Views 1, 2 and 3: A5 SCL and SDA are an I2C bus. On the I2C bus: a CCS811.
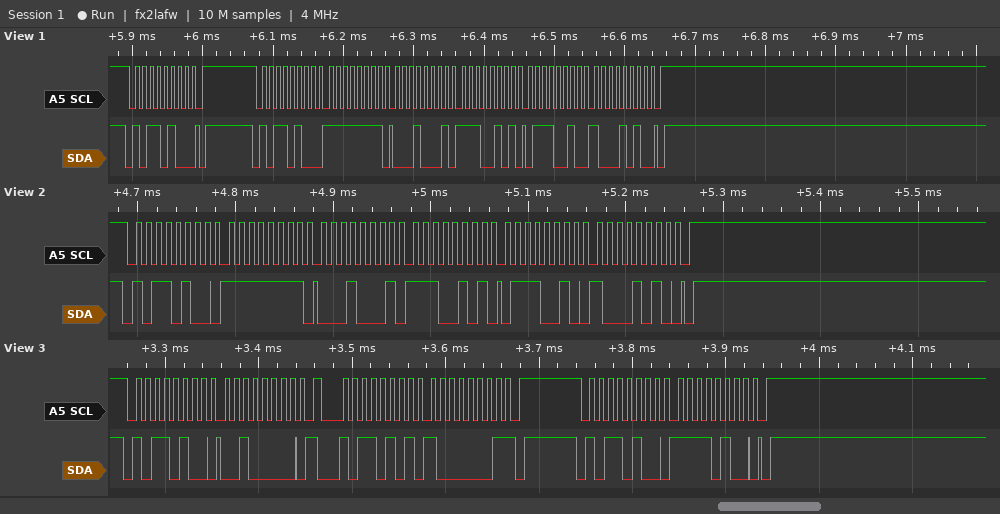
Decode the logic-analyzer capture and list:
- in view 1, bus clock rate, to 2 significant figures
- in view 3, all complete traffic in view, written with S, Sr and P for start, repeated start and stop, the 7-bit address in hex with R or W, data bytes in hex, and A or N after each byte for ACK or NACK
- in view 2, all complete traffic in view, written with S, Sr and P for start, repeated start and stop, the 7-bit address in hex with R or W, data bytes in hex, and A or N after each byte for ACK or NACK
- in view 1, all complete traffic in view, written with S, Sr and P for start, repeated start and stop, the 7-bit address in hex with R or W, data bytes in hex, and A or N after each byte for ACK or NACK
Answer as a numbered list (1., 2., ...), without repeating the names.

1. 100 kHz
2. S 5AW A 20 A Sr 5AR A 81 N P S 5AW A F4 A P
3. S 5AW A FF A 11 A E5 A 72 A 8A A P
4. S 5AW A P S 5AW A FF A 11 A E5 A 72 A 8A A P
